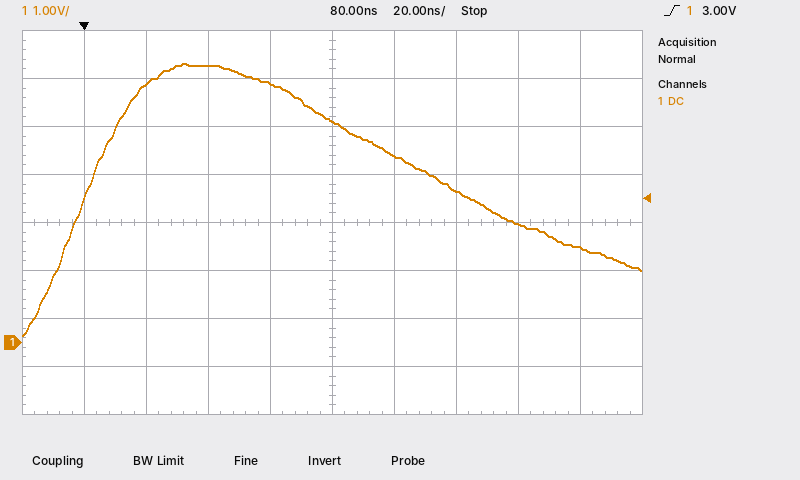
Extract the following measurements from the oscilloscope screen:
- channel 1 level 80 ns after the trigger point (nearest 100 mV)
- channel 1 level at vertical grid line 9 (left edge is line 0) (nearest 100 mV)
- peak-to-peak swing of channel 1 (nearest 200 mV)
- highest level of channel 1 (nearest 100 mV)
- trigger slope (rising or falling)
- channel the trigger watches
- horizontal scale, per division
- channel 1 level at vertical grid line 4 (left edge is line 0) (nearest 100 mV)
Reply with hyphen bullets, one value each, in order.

- 4.6 V
- 2.0 V
- 5.6 V
- 5.8 V
- rising
- channel 1
- 20 ns
- 5.4 V
